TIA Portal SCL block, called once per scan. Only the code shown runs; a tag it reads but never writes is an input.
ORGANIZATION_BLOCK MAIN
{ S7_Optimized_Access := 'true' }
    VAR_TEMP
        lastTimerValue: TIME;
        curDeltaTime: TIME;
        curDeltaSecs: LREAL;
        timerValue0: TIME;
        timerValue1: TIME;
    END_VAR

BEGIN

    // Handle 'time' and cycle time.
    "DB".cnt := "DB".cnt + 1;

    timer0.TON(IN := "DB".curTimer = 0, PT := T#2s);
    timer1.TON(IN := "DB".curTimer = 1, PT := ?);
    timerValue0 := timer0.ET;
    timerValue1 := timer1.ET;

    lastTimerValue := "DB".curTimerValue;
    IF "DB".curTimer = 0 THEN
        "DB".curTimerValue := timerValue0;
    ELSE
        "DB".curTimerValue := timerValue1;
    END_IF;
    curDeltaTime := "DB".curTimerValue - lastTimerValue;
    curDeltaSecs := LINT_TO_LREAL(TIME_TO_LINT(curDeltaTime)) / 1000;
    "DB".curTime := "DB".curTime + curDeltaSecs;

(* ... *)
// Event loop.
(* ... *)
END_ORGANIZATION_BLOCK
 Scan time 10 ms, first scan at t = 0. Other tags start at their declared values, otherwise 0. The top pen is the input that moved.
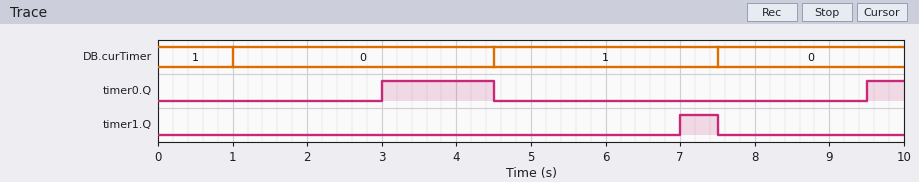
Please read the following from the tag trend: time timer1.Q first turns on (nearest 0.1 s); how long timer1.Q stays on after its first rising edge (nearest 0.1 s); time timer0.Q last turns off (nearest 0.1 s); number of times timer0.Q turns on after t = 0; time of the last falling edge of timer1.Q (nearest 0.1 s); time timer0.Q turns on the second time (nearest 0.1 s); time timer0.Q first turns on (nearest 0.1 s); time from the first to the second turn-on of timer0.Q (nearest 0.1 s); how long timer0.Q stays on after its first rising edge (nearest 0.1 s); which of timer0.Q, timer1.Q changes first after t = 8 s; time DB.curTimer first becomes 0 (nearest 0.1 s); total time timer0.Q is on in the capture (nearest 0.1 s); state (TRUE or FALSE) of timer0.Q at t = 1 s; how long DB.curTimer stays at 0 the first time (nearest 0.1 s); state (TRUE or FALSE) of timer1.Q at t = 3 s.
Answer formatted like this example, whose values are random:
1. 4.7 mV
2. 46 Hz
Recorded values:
1. 7.0 s
2. 0.5 s
3. 4.5 s
4. 2
5. 7.5 s
6. 9.5 s
7. 3.0 s
8. 6.5 s
9. 1.5 s
10. timer0.Q
11. 1.0 s
12. 2.0 s
13. FALSE
14. 3.5 s
15. FALSE
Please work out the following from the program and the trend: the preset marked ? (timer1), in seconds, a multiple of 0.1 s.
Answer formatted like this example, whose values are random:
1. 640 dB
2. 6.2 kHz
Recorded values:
1. 2.5 s
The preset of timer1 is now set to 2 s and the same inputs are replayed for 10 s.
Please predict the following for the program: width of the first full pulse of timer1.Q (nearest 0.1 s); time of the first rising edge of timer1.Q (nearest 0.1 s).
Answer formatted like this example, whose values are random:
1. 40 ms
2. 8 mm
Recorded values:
1. 1.0 s
2. 6.5 s
